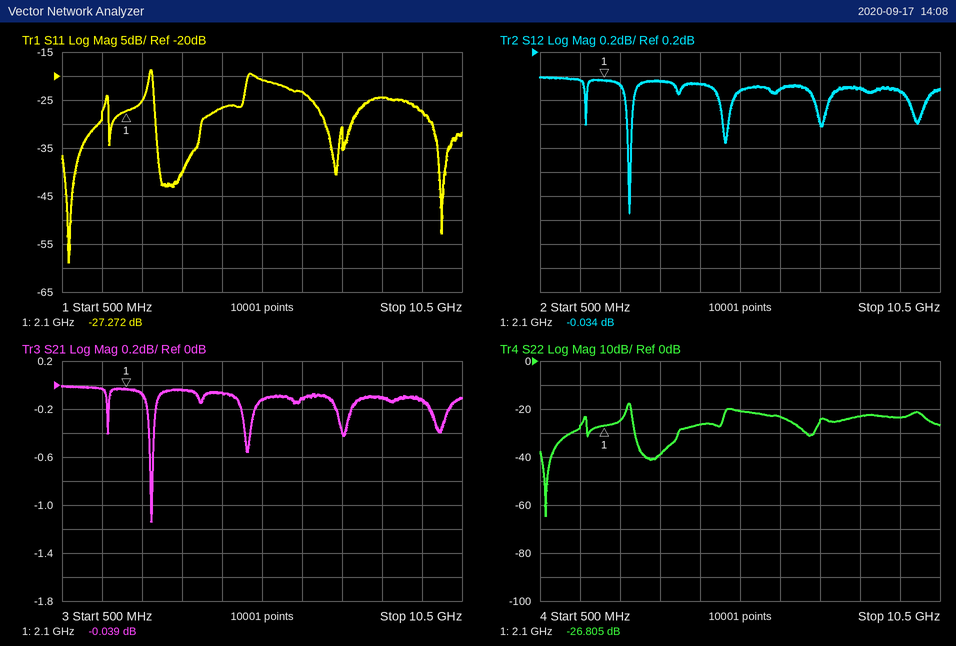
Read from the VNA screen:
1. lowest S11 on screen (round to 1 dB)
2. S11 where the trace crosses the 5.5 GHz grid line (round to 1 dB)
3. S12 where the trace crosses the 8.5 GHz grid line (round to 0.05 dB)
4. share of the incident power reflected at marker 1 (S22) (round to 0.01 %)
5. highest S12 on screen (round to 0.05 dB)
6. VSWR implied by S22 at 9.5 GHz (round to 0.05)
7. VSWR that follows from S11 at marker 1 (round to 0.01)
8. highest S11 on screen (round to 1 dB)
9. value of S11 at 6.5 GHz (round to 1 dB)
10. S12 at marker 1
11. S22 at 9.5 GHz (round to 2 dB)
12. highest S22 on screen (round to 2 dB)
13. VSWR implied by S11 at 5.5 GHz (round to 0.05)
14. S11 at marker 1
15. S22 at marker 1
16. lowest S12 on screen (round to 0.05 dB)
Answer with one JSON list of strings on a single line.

["-59 dB", "-21 dB", "-0.10 dB", "0.21 %", "0.00 dB", "1.15", "1.09", "-19 dB", "-23 dB", "-0.034 dB", "-24 dB", "-18 dB", "1.20", "-27.272 dB", "-26.805 dB", "-1.15 dB"]
